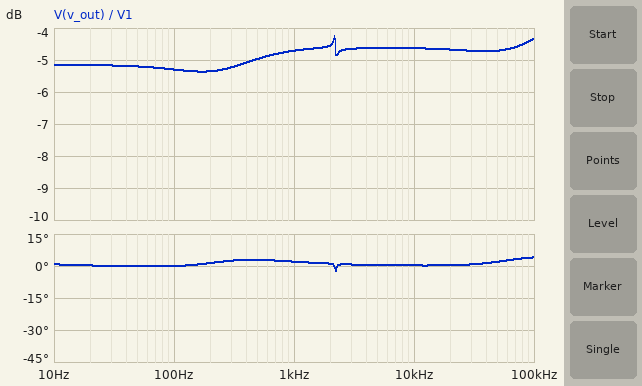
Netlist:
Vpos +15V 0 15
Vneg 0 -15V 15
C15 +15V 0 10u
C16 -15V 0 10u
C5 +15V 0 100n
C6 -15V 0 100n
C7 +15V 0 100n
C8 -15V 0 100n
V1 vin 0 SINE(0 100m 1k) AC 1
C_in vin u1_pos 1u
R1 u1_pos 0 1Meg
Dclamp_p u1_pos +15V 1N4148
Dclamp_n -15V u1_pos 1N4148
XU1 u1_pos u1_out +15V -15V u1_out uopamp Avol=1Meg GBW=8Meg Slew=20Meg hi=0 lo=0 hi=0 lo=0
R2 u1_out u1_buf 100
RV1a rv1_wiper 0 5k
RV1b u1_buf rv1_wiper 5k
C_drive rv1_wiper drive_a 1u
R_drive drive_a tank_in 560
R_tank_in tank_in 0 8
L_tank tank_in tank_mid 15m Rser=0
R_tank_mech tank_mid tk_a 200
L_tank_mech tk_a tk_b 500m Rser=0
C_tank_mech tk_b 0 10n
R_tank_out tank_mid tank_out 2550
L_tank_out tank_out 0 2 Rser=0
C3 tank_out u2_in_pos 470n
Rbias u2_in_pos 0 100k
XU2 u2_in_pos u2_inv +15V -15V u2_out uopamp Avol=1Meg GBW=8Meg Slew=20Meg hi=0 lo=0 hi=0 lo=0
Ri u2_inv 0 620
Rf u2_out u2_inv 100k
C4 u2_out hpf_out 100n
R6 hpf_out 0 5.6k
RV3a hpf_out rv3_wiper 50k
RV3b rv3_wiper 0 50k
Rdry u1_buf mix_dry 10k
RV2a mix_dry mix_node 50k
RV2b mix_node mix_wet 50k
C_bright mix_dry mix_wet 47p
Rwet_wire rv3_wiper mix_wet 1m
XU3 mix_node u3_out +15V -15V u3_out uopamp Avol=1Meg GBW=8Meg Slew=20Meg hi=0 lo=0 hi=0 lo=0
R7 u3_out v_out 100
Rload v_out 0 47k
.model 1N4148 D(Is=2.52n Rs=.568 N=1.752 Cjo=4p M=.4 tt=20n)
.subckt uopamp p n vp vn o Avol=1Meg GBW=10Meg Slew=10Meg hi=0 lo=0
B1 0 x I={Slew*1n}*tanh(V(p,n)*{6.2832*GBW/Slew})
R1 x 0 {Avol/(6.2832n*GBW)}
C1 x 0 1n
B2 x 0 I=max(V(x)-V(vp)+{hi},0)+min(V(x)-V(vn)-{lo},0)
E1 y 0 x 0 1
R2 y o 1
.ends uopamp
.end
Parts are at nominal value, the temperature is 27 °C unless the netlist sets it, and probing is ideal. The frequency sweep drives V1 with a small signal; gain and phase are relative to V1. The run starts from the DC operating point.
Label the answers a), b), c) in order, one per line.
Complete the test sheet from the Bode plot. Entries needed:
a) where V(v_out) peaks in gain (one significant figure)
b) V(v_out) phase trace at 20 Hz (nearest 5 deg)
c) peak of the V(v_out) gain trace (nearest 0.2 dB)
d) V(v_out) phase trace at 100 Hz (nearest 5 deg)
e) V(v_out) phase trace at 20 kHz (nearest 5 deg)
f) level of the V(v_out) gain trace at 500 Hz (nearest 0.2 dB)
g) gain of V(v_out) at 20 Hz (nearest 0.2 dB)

a) 2 kHz
b) 0 deg
c) -4.2 dB
d) 0 deg
e) 0 deg
f) -5.0 dB
g) -5.2 dB
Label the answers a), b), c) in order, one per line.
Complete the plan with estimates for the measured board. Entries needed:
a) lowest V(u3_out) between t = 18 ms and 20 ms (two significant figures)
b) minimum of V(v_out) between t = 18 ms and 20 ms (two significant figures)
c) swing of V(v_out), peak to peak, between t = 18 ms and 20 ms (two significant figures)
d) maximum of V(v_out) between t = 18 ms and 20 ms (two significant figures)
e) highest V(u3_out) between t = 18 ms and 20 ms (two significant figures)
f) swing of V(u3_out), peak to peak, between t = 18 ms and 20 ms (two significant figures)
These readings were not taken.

a) -58 mV
b) -58 mV
c) 120 mV
d) 58 mV
e) 58 mV
f) 120 mV
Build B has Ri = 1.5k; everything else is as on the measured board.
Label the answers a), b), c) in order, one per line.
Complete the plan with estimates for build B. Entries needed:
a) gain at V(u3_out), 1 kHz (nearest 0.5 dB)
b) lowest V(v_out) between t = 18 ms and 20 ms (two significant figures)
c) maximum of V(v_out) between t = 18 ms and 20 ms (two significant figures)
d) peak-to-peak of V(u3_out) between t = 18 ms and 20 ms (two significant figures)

a) -5.0 dB
b) -56 mV
c) 56 mV
d) 110 mV
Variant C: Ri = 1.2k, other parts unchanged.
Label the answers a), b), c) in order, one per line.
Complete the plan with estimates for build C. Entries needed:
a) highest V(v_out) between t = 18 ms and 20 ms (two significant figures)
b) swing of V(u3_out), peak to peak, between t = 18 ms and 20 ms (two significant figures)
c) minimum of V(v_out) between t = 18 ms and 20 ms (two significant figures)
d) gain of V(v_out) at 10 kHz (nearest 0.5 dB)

a) 56 mV
b) 110 mV
c) -56 mV
d) -5.0 dB
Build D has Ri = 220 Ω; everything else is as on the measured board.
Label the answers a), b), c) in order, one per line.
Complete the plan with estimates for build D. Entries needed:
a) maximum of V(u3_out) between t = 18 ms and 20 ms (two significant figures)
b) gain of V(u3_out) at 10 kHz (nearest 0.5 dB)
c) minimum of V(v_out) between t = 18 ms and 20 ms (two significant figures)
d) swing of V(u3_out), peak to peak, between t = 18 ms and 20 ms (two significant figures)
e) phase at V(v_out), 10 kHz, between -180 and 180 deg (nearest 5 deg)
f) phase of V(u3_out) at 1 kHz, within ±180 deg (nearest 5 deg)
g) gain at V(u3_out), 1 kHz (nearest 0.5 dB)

a) 65 mV
b) -4.0 dB
c) -65 mV
d) 130 mV
e) -5 deg
f) 5 deg
g) -3.5 dB
